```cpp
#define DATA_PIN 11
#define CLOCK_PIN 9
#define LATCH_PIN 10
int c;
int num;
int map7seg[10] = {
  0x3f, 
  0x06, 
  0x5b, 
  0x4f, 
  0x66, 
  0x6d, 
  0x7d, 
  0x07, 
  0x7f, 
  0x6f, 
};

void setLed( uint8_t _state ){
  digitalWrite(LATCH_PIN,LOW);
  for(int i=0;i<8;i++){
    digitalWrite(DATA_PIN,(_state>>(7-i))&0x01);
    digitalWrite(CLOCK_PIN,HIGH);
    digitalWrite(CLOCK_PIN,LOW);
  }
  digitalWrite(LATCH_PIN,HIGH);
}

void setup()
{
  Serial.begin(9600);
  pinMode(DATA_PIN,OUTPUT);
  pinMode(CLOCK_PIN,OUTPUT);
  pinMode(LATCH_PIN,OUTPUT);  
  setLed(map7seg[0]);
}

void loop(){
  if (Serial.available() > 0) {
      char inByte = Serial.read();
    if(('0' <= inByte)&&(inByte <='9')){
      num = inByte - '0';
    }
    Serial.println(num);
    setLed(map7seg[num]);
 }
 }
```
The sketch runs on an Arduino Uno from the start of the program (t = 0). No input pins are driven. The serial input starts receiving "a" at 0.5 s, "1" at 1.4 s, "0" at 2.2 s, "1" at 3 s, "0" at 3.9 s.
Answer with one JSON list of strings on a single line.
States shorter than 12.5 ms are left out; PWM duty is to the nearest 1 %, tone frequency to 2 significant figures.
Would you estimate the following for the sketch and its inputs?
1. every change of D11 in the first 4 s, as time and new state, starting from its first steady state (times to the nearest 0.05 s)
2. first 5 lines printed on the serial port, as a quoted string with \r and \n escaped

["0 s high; 1.4 s low; 2.2 s high; 3 s low; 3.9 s high", "\"0\\r\\n1\\r\\n0\\r\\n1\\r\\n0\\r\\n\""]
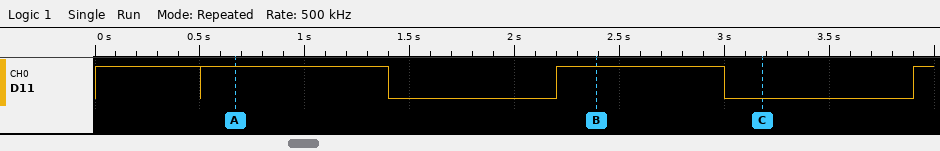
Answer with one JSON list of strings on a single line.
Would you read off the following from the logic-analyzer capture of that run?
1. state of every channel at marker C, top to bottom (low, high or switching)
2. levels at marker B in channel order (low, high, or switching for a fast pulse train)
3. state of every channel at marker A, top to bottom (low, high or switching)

["D11 low", "D11 high", "D11 high"]
